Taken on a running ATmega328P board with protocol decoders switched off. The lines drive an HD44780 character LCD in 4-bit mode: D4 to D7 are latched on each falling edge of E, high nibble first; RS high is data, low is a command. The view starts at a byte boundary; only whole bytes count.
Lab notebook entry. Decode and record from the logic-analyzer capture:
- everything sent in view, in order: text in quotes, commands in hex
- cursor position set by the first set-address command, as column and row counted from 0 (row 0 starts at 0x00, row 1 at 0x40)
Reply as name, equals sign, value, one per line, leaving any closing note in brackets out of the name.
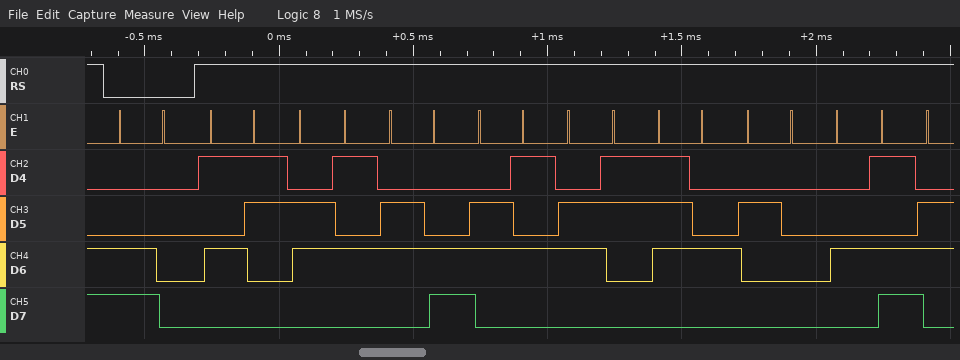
everything sent in view, in order: text in quotes, commands in hex = 0xC0 "Select M"
cursor position set by the first set-address command, as column and row counted from 0 = column 0, row 1
